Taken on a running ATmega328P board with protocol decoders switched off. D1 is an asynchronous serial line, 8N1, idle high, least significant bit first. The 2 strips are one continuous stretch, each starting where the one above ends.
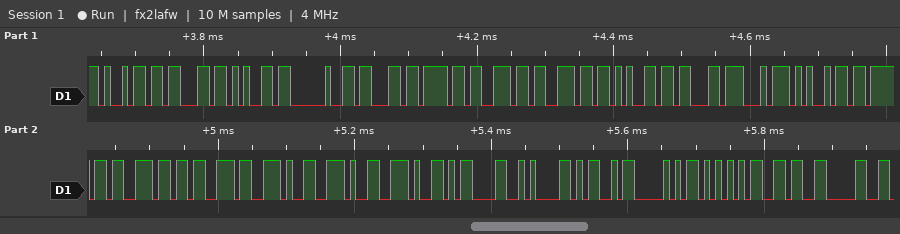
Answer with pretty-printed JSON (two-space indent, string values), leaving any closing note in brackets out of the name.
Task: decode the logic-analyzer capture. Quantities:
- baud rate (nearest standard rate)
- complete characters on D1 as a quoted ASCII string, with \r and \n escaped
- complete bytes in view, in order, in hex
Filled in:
{
  "baud rate": "115200 baud",
  "complete characters on D1 as a quoted ASCII string, with \\r and \\n escaped": "\"ice connections...\\r\\nMPU60\"",
  "complete bytes in view, in order, in hex": "69 63 65 20 63 6F 6E 6E 65 63 74 69 6F 6E 73 2E 2E 2E 0D 0A 4D 50 55 36 30"
}
